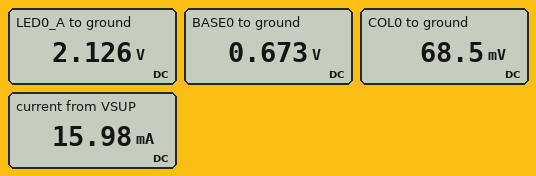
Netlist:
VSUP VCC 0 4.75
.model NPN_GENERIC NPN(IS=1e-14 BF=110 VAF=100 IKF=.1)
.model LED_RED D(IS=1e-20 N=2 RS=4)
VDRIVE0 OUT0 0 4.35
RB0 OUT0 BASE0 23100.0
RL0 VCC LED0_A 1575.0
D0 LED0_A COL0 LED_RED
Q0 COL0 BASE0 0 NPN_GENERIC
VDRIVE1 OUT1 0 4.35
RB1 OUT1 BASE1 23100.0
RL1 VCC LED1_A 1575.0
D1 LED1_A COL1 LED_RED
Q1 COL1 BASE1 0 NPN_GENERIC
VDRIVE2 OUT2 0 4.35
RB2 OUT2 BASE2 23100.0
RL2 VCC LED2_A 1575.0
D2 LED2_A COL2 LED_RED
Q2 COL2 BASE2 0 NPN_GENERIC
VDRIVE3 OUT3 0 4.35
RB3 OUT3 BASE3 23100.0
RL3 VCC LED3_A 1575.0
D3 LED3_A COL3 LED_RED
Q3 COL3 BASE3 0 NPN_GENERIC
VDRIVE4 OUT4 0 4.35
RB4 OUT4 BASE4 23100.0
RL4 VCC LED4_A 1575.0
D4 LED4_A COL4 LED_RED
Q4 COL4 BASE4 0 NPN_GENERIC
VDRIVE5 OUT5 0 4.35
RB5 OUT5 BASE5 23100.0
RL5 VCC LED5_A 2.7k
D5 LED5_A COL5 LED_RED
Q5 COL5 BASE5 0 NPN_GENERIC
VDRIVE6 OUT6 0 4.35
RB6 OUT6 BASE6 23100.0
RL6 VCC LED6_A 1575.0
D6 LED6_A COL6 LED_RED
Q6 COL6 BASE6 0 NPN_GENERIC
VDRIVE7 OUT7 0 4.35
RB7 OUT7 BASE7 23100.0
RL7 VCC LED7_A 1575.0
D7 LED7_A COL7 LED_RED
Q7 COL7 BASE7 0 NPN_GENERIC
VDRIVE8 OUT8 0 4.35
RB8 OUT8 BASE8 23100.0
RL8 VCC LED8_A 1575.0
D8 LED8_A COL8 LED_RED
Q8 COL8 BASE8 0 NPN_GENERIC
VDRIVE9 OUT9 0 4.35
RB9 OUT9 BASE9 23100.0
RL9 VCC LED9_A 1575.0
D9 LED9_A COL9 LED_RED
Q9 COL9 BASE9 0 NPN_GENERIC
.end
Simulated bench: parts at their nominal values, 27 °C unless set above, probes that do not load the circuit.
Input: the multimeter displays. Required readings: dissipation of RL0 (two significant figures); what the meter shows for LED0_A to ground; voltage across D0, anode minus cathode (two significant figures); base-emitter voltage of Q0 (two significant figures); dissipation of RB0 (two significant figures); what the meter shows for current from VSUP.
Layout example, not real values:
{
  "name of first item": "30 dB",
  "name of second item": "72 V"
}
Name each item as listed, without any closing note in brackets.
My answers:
{
  "dissipation of RL0": "4.4 mW",
  "what the meter shows for LED0_A to ground": "2.126 V",
  "voltage across D0, anode minus cathode": "2.1 V",
  "base-emitter voltage of Q0": "670 mV",
  "dissipation of RB0": "590 µW",
  "what the meter shows for current from VSUP": "15.98 mA"
}
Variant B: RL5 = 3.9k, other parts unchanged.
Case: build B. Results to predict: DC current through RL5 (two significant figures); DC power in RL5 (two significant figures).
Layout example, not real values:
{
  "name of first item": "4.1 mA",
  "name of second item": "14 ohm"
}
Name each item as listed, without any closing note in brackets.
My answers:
{
  "DC current through RL5": "690 µA",
  "DC power in RL5": "1.9 mW"
}
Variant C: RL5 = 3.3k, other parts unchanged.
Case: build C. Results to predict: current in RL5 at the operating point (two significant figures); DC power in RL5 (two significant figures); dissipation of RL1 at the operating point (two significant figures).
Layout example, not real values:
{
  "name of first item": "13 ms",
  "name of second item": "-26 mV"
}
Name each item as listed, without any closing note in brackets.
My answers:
{
  "current in RL5 at the operating point": "810 µA",
  "DC power in RL5": "2.2 mW",
  "dissipation of RL1 at the operating point": "4.4 mW"
}
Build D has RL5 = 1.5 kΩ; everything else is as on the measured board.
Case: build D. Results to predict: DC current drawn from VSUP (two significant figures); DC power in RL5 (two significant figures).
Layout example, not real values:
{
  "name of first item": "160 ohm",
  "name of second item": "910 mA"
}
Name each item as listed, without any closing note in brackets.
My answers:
{
  "DC current drawn from VSUP": "17 mA",
  "DC power in RL5": "4.6 mW"
}
